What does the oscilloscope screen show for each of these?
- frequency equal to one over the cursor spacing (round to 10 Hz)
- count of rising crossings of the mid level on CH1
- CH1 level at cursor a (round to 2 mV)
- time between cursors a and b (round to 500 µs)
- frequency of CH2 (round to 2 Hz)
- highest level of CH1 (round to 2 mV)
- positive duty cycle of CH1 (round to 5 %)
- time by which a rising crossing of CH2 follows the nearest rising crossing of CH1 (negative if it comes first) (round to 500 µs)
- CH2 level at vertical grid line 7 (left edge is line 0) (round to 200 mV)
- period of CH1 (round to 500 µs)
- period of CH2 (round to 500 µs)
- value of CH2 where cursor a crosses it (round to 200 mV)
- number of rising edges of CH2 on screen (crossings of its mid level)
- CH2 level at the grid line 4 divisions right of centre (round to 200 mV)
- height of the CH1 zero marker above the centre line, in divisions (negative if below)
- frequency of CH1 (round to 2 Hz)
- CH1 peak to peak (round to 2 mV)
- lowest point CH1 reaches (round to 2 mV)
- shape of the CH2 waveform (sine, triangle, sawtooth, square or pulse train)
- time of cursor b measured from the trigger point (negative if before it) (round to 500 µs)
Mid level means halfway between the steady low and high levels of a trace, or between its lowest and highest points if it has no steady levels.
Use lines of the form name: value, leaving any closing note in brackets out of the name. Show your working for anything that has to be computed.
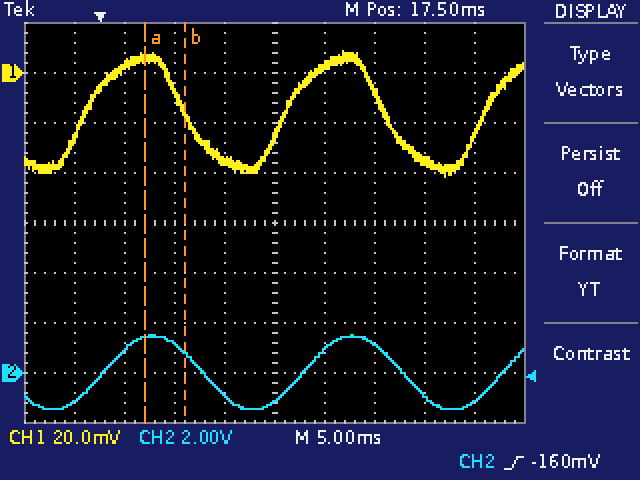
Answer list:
frequency equal to one over the cursor spacing: 1 / 4.0 ms ≈ 250 Hz
count of rising crossings of the mid level on CH1: 3
CH1 level at cursor a: 6 mV
time between cursors a and b: 4.0 ms
frequency of CH2: 1 / 20.0 ms ≈ 50 Hz
highest level of CH1: 8 mV
positive duty cycle of CH1: 50 %
time by which a rising crossing of CH2 follows the nearest rising crossing of CH1 (negative if it comes first): +2.0 ms
CH2 level at vertical grid line 7 (left edge is line 0): 1.2 V
period of CH1: 20.0 ms
period of CH2: 20.0 ms
value of CH2 where cursor a crosses it: 1.4 V
number of rising edges of CH2 on screen: 3
CH2 level at the grid line 4 divisions right of centre: -1.2 V
height of the CH1 zero marker above the centre line, in divisions: +3.0 div
frequency of CH1: 1 / 20.0 ms ≈ 50 Hz
CH1 peak to peak: 8 mV − (-42 mV) = 50 mV
lowest point CH1 reaches: -42 mV
shape of the CH2 waveform: sine
time of cursor b measured from the trigger point (negative if before it): +8.5 ms
